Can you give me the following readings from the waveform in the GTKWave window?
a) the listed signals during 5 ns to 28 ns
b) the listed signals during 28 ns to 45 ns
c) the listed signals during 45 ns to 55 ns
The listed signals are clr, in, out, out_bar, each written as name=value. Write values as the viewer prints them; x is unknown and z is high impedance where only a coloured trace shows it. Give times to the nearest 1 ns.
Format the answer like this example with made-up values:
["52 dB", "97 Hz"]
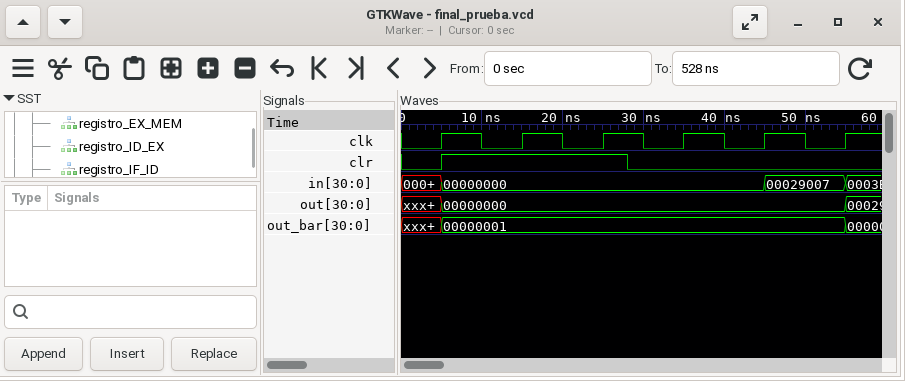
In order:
["clr=1, in=00000000, out=00000000, out_bar=00000001", "clr=0, in=00000000, out=00000000, out_bar=00000001", "clr=0, in=00029007, out=00000000, out_bar=00000001"]
